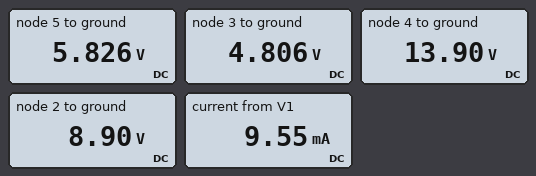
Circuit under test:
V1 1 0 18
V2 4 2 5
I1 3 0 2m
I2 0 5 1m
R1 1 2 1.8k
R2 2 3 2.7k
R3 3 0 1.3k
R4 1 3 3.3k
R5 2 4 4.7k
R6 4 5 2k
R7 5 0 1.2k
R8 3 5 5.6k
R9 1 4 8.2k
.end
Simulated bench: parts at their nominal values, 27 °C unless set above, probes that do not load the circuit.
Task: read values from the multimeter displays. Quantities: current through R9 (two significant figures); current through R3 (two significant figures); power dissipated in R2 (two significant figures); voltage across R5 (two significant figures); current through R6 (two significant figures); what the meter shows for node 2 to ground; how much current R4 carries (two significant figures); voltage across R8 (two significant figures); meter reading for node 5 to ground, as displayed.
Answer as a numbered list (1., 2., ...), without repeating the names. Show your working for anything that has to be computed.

1. (18 V - 13.9 V) / 8.2 kΩ = 500 µA
2. (4.806 V) / 1.3 kΩ = 3.7 mA
3. (8.9 V - 4.806 V)^2 / 2.7 kΩ = 6.2 mW
4. 13.9 V - 8.9 V = 5.0 V
5. (13.9 V - 5.826 V) / 2 kΩ = 4.0 mA
6. 8.90 V
7. (18 V - 4.806 V) / 3.3 kΩ = 4.0 mA
8. 5.826 V - 4.806 V = 1.0 V
9. 5.826 V
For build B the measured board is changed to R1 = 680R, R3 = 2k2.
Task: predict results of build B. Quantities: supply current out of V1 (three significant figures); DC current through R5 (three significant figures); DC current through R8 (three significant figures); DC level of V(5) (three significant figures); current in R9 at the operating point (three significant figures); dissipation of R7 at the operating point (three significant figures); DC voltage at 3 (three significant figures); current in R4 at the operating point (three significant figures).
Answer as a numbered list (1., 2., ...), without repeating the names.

1. 10.6 mA
2. 1.06 mA
3. 23.3 µA
4. 7.48 V
5. 133 nA
6. 46.7 mW
7. 7.35 V
8. 3.23 mA
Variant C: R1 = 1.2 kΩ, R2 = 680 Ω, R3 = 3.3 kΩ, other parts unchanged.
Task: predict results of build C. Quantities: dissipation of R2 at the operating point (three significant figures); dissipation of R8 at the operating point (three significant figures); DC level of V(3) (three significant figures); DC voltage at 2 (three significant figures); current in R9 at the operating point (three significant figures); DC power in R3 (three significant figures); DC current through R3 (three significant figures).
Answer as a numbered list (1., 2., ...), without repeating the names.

1. 3.59 mW
2. 761 µW
3. 8.88 V
4. 10.4 V
5. 312 µA
6. 23.9 mW
7. 2.69 mA
